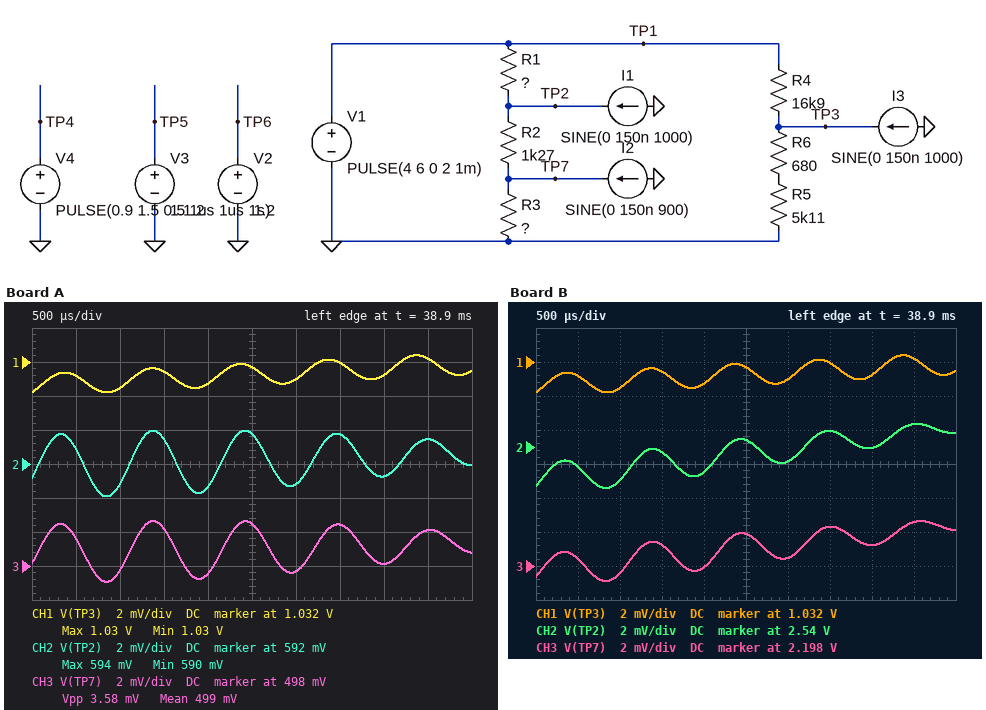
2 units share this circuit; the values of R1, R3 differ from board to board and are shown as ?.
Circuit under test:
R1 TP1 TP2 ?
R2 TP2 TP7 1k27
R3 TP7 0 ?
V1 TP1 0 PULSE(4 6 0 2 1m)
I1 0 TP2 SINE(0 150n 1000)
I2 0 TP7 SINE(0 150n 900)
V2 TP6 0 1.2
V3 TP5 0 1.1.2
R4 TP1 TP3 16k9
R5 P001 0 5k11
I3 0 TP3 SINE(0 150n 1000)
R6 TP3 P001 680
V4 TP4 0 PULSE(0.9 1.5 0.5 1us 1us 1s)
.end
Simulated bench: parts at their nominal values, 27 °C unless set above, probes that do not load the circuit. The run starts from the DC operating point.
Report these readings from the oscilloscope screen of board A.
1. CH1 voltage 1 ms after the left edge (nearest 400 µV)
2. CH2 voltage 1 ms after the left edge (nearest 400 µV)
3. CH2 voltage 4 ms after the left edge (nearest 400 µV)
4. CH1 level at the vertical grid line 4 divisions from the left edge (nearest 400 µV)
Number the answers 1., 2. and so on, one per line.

1. 1.0304 V
2. 590.8 mV
3. 591.2 mV
4. 1.0308 V
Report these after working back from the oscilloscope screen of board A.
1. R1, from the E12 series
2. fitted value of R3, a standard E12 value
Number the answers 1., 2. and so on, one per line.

1. 47 kΩ
2. 6.8 kΩ
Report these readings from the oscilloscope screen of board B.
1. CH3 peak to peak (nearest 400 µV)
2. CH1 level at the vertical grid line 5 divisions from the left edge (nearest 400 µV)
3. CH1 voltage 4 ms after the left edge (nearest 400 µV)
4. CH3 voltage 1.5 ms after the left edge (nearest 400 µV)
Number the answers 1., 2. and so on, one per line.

1. 3.6 mV
2. 1.0316 V
3. 1.0312 V
4. 2.1992 V
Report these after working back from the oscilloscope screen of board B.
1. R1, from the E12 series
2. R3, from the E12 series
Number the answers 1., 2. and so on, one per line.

1. 5.6 kΩ
2. 8.2 kΩ
